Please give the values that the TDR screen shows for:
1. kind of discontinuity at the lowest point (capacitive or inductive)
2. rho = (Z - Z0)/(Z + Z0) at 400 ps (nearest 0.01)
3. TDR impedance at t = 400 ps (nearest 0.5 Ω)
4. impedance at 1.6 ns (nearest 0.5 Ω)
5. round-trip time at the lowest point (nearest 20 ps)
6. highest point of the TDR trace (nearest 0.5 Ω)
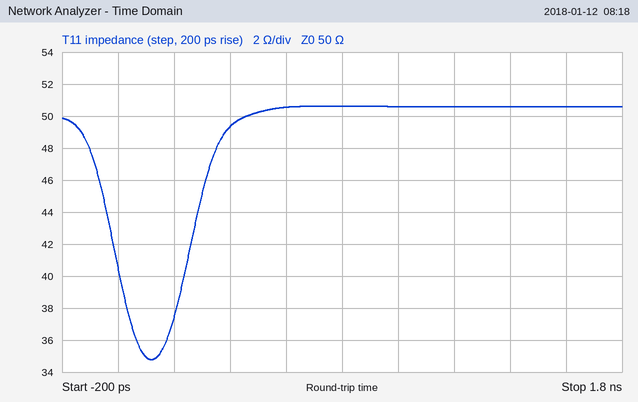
capacitive
-0.01
49.5 Ω
50.5 Ω
120 ps
50.5 Ω
